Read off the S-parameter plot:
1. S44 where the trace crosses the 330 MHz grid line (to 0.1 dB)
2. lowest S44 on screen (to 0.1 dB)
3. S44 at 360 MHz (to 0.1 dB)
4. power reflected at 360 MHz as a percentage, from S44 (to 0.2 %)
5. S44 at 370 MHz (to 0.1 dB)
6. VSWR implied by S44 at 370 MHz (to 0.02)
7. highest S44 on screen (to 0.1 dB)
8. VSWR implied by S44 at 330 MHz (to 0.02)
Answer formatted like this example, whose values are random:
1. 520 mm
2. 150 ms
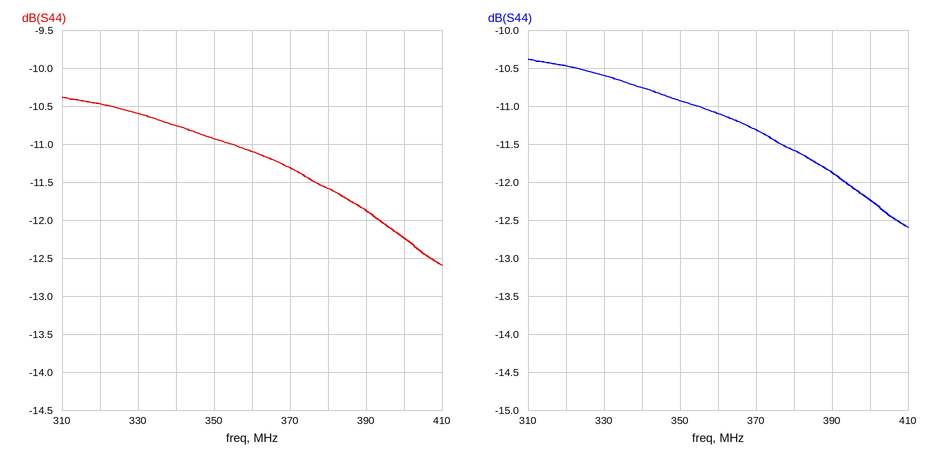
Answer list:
1. -10.6 dB
2. -12.6 dB
3. -11.1 dB
4. 7.8 %
5. -11.3 dB
6. 1.74
7. -10.4 dB
8. 1.84
